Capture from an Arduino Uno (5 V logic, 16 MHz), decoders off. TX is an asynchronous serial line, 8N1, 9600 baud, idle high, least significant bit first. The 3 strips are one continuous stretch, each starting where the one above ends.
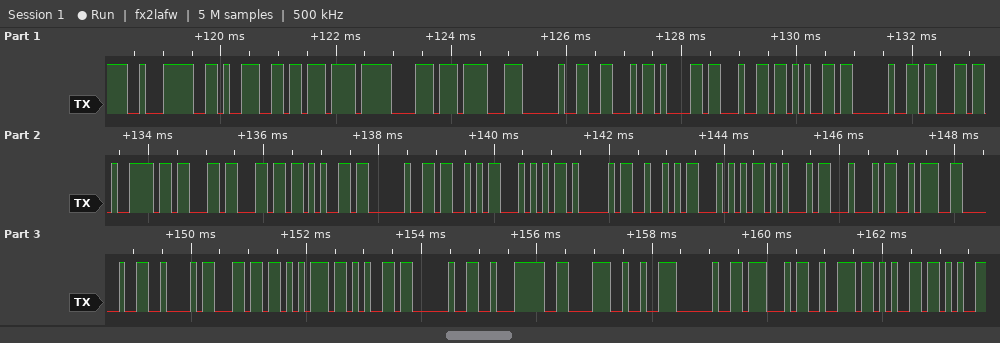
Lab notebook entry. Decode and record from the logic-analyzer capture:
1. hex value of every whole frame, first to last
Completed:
E2 96 B6 EF B8 8F 20 46 61 64 65 20 63 79 63 6C 65 20 53 54 41 52 54 45 44 3A 20 42 6C 75 65 20 E2 86 92 20 47 72 65
